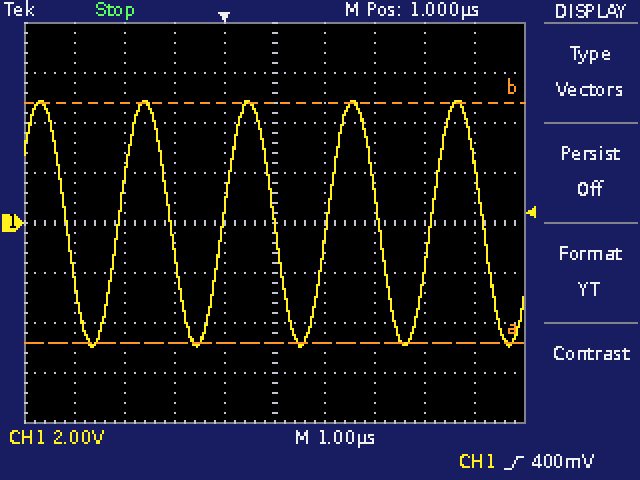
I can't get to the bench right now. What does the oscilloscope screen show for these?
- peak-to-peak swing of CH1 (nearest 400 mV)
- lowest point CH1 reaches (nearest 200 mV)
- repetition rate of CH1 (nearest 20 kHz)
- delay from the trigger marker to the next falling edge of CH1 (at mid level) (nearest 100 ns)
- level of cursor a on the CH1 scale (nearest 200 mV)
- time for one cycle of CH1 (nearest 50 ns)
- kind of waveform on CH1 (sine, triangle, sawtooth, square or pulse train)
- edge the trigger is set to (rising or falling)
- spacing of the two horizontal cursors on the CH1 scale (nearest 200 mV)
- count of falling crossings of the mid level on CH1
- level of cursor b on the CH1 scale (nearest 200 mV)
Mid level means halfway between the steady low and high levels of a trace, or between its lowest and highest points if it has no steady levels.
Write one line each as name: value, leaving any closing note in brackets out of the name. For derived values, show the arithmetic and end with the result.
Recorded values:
peak-to-peak swing of CH1: 10.0 V
lowest point CH1 reaches: -5.0 V
repetition rate of CH1: 1 / 2.10 µs ≈ 476 kHz, so 480 kHz to the nearest 20 kHz
delay from the trigger marker to the next falling edge of CH1 (at mid level): 1.0 µs
level of cursor a on the CH1 scale: -4.8 V
time for one cycle of CH1: 2.10 µs
kind of waveform on CH1: sine
edge the trigger is set to: rising
spacing of the two horizontal cursors on the CH1 scale: 9.6 V
count of falling crossings of the mid level on CH1: 5
level of cursor b on the CH1 scale: 4.8 V
